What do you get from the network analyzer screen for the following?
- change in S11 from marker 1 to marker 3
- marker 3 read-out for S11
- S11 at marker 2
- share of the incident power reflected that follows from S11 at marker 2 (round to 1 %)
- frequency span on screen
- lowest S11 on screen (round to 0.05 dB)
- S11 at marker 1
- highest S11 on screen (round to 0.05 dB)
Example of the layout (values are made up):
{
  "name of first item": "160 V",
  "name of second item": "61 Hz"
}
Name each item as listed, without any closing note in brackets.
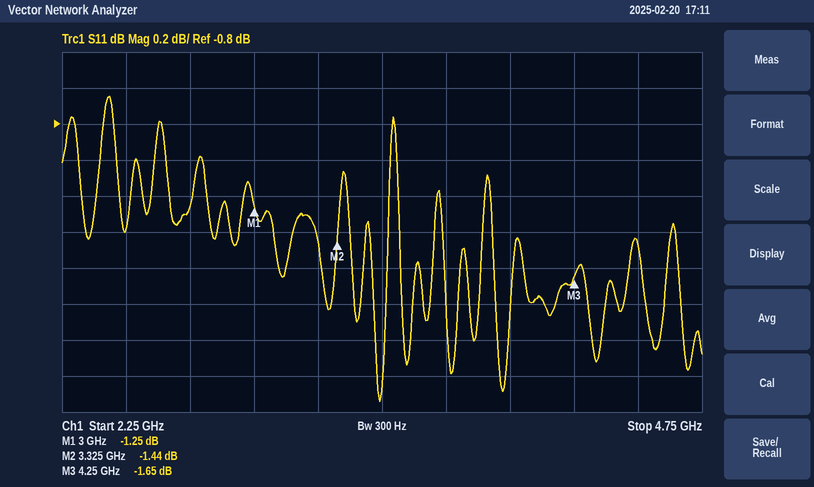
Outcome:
{
  "change in S11 from marker 1 to marker 3": "-0.40 dB",
  "marker 3 read-out for S11": "-1.65 dB",
  "S11 at marker 2": "-1.44 dB",
  "share of the incident power reflected that follows from S11 at marker 2": "72 %",
  "frequency span on screen": "2.5 GHz",
  "lowest S11 on screen": "-2.35 dB",
  "S11 at marker 1": "-1.25 dB",
  "highest S11 on screen": "-0.65 dB"
}
